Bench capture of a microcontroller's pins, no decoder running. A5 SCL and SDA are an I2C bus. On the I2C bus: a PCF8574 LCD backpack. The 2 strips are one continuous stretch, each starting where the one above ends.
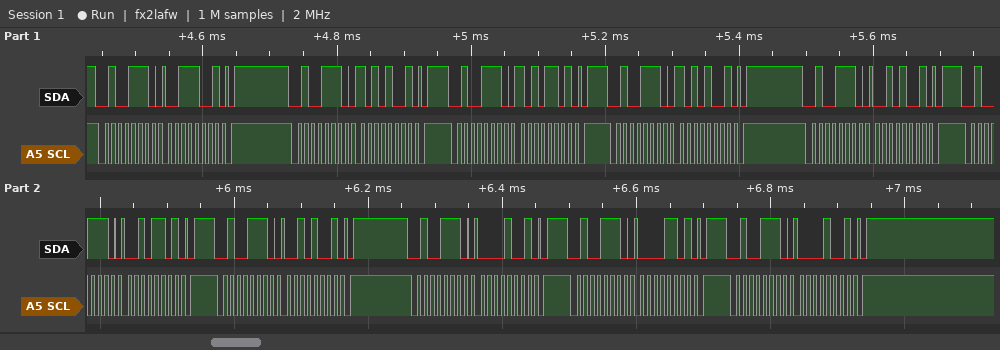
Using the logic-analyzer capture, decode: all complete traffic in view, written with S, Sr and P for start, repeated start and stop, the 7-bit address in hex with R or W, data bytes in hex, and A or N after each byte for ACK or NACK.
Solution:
S 27W A 39 A P S 27W A A9 A P S 27W A AD A P S 27W A A9 A P S 27W A 29 A P S 27W A 2D A P S 27W A 29 A P S 27W A 09 A P S 27W A 0D A P S 27W A 09 A P
